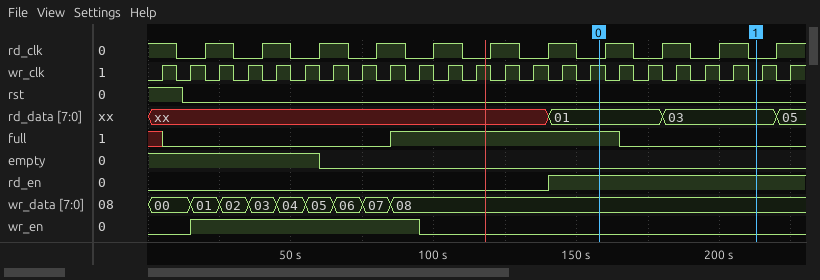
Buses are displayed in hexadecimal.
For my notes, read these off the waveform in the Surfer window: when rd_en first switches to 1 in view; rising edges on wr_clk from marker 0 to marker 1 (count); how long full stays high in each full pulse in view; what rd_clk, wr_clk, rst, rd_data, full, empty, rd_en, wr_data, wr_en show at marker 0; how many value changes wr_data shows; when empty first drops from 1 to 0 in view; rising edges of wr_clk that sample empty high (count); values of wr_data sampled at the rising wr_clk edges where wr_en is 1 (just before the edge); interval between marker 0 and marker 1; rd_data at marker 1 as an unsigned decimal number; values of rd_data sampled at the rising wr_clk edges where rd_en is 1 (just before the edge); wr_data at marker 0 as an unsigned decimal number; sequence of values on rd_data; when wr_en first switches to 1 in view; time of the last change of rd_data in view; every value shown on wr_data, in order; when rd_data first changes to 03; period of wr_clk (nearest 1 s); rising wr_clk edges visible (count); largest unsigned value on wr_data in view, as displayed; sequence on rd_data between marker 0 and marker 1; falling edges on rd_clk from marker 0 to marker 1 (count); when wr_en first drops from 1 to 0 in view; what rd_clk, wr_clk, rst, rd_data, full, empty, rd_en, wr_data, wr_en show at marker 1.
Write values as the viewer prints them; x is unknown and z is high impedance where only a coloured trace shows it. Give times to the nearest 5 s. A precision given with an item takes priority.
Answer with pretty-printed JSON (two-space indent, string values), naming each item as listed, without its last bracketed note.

{
  "when rd_en first switches to 1 in view": "140 s",
  "rising edges on wr_clk from marker 0 to marker 1": "5",
  "how long full stays high in each full pulse in view": "80 s",
  "what rd_clk, wr_clk, rst, rd_data, full, empty, rd_en, wr_data, wr_en show at marker 0": "rd_clk=0, wr_clk=1, rst=0, rd_data=01, full=1, empty=0, rd_en=1, wr_data=08, wr_en=0",
  "how many value changes wr_data shows": "8",
  "when empty first drops from 1 to 0 in view": "60 s",
  "rising edges of wr_clk that sample empty high": "6",
  "values of wr_data sampled at the rising wr_clk edges where wr_en is 1": "01, 02, 03, 04, 05, 06, 07, 08",
  "interval between marker 0 and marker 1": "55 s",
  "rd_data at marker 1 as an unsigned decimal number": "3",
  "values of rd_data sampled at the rising wr_clk edges where rd_en is 1": "01, 01, 01, 01, 03, 03, 03, 03, 05",
  "wr_data at marker 0 as an unsigned decimal number": "8",
  "sequence of values on rd_data": "xx, 01, 03, 05",
  "when wr_en first switches to 1 in view": "15 s",
  "time of the last change of rd_data in view": "220 s",
  "every value shown on wr_data, in order": "00, 01, 02, 03, 04, 05, 06, 07, 08",
  "when rd_data first changes to 03": "180 s",
  "period of wr_clk": "10 s",
  "rising wr_clk edges visible": "23",
  "largest unsigned value on wr_data in view, as displayed": "08",
  "sequence on rd_data between marker 0 and marker 1": "01, 03",
  "falling edges on rd_clk from marker 0 to marker 1": "3",
  "when wr_en first drops from 1 to 0 in view": "95 s",
  "what rd_clk, wr_clk, rst, rd_data, full, empty, rd_en, wr_data, wr_en show at marker 1": "rd_clk=0, wr_clk=0, rst=0, rd_data=03, full=0, empty=0, rd_en=1, wr_data=08, wr_en=0"
}
